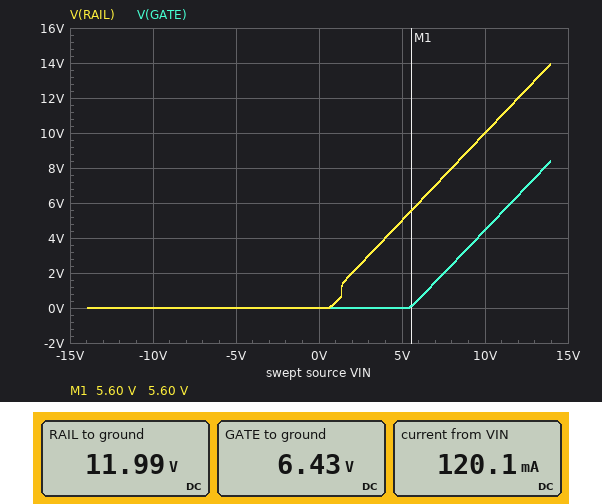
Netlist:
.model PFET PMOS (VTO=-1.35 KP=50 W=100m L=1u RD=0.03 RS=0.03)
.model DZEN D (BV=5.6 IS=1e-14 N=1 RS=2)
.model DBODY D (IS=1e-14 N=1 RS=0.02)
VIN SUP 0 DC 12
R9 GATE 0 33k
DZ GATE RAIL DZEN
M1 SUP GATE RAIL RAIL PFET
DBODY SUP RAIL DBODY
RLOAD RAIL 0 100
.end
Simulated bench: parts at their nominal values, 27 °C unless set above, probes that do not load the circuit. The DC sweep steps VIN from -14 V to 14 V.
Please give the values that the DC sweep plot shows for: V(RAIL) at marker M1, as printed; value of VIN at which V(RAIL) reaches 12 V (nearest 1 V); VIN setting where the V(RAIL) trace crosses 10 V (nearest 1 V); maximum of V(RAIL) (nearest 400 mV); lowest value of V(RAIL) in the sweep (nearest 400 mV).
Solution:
5.60 V
12 V
10 V
14.0 V
0 V
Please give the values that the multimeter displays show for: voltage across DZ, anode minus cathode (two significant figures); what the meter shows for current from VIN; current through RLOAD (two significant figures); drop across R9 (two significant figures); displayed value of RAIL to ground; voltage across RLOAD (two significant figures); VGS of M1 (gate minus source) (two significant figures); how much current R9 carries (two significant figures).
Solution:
-5.6 V
120.1 mA
120 mA
6.4 V
11.99 V
12 V
-5.6 V
190 µA
